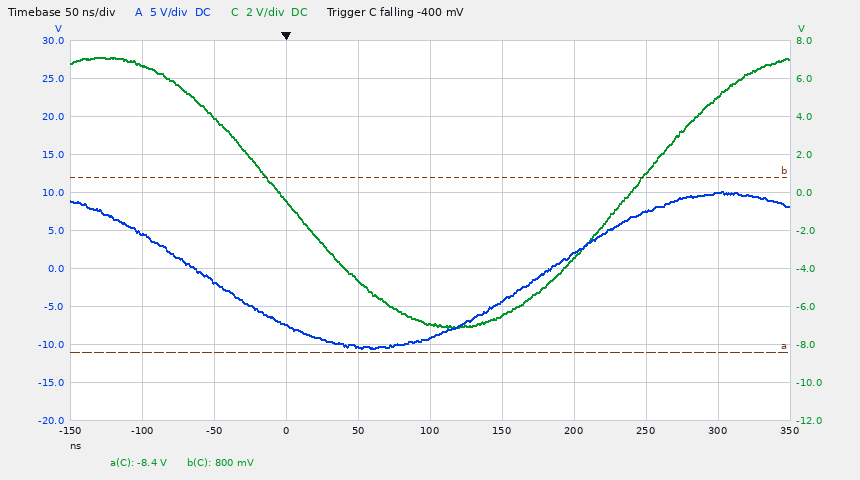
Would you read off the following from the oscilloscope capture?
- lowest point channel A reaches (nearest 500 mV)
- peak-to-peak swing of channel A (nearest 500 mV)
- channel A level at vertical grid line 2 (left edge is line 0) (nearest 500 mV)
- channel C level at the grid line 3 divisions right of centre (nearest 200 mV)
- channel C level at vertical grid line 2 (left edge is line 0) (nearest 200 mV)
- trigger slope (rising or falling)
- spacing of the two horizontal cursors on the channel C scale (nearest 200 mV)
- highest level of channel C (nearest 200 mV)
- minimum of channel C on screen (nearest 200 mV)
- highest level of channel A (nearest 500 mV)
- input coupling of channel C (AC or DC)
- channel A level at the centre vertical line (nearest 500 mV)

-10.5 V
20.5 V
-1.5 V
1.0 V
4.0 V
falling
9.2 V
7.2 V
-7.2 V
10.0 V
DC
-9.0 V
